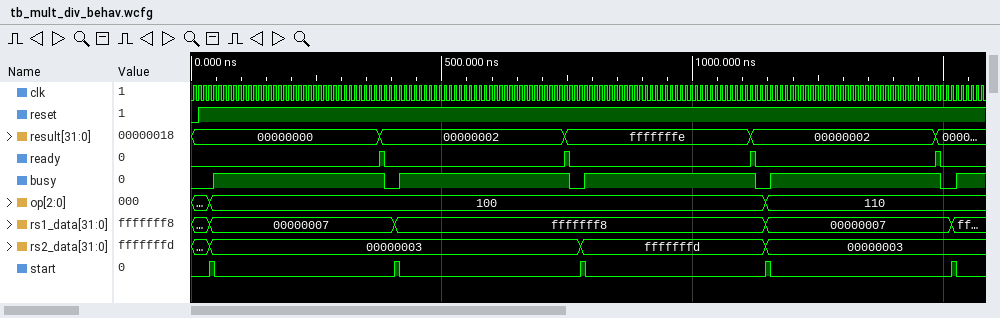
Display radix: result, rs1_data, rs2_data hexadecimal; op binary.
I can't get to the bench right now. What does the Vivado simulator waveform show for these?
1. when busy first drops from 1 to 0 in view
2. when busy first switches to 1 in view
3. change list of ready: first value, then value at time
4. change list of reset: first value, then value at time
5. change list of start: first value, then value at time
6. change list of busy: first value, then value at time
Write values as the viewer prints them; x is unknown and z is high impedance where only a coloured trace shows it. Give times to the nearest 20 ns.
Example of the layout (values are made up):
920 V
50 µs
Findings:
380 ns
40 ns
0, 1 at 380 ns, 0 at 380 ns, 1 at 740 ns, 0 at 760 ns, 1 at 1120 ns, 0 at 1120 ns, 1 at 1480 ns, 0 at 1500 ns
0, 1 at 20 ns
0, 1 at 40 ns, 0 at 40 ns, 1 at 400 ns, 0 at 420 ns, 1 at 780 ns, 0 at 780 ns, 1 at 1140 ns, 0 at 1160 ns, 1 at 1520 ns, 0 at 1520 ns
0, 1 at 40 ns, 0 at 380 ns, 1 at 420 ns, 0 at 760 ns, 1 at 780 ns, 0 at 1120 ns, 1 at 1160 ns, 0 at 1500 ns, 1 at 1520 ns
